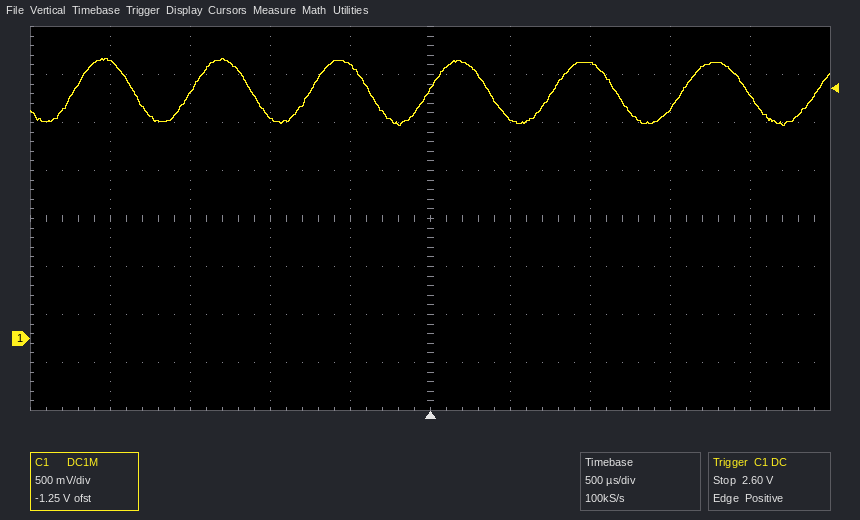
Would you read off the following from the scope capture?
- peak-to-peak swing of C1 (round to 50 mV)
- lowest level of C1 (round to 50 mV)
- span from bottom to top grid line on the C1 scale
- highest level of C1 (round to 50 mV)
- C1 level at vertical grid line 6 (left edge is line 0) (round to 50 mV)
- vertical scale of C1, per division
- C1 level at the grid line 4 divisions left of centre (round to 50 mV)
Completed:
700 mV
2.20 V
4 V
2.90 V
2.30 V
500 mV
2.90 V
